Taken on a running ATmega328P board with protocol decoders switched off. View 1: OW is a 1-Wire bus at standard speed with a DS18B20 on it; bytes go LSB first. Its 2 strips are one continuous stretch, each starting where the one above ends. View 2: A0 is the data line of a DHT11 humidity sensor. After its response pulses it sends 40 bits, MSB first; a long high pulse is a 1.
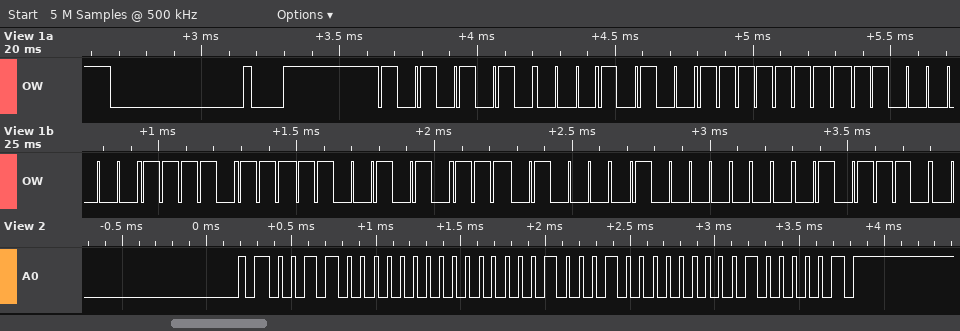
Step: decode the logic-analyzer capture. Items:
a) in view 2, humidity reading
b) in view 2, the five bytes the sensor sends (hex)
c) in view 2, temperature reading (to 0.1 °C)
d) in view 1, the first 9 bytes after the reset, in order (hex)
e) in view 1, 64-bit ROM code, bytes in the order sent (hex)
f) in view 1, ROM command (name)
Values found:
48 %
30 00 11 00 41
17.0 °C
55 28 FF 03 EF 53 17 02 74
28 FF 03 EF 53 17 02 74
Match ROM
